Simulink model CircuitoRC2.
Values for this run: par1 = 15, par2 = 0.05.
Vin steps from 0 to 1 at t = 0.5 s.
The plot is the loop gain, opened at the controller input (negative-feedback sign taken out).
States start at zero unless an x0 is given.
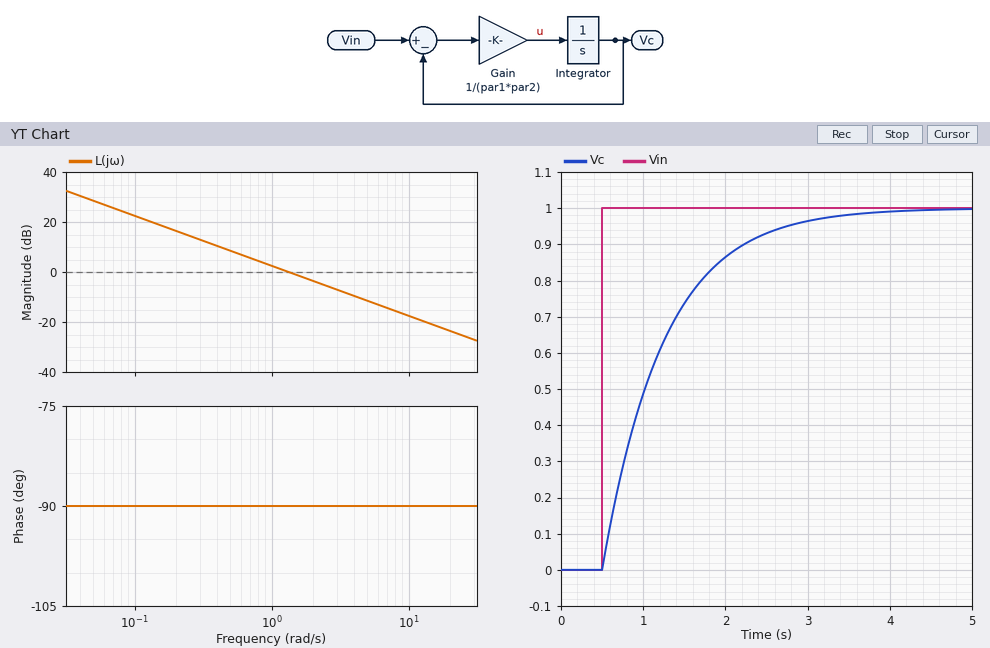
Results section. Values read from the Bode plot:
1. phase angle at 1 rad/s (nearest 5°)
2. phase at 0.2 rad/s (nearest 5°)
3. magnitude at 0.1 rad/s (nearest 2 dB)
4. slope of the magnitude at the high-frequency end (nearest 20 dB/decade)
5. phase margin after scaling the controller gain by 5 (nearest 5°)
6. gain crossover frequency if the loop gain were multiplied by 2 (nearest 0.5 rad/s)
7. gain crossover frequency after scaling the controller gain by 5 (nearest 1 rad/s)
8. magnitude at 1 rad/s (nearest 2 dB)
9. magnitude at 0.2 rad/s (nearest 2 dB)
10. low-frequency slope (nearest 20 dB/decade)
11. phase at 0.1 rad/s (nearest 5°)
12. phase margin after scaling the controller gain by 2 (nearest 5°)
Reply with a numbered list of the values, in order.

1. -90°
2. -90°
3. 22 dB
4. -20 dB/decade
5. 90°
6. 2.5 rad/s
7. 7 rad/s
8. 2 dB
9. 16 dB
10. -20 dB/decade
11. -90°
12. 90°
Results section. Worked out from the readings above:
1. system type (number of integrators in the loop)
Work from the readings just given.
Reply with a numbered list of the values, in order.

1. 1
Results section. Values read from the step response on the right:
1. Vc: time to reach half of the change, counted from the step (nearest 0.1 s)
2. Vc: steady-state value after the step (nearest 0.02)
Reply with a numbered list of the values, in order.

1. 0.5 s
2. 1.00
